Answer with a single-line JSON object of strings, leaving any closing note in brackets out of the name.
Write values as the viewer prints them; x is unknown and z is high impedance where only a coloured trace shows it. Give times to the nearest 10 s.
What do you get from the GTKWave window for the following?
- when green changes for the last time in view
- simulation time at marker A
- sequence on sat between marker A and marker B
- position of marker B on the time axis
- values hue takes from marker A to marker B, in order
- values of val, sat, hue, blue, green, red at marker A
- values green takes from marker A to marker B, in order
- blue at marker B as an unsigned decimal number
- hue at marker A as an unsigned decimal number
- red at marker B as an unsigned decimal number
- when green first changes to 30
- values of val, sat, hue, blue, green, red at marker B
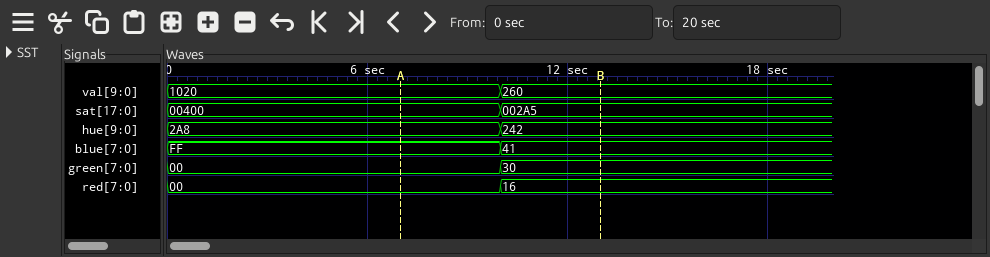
{"when green changes for the last time in view": "10 s", "simulation time at marker A": "10 s", "sequence on sat between marker A and marker B": "00400, 002A5", "position of marker B on the time axis": "10 s", "values hue takes from marker A to marker B, in order": "2A8, 242", "values of val, sat, hue, blue, green, red at marker A": "val=1020, sat=00400, hue=2A8, blue=FF, green=00, red=00", "values green takes from marker A to marker B, in order": "00, 30", "blue at marker B as an unsigned decimal number": "65", "hue at marker A as an unsigned decimal number": "680", "red at marker B as an unsigned decimal number": "22", "when green first changes to 30": "10 s", "values of val, sat, hue, blue, green, red at marker B": "val=260, sat=002A5, hue=242, blue=41, green=30, red=16"}
